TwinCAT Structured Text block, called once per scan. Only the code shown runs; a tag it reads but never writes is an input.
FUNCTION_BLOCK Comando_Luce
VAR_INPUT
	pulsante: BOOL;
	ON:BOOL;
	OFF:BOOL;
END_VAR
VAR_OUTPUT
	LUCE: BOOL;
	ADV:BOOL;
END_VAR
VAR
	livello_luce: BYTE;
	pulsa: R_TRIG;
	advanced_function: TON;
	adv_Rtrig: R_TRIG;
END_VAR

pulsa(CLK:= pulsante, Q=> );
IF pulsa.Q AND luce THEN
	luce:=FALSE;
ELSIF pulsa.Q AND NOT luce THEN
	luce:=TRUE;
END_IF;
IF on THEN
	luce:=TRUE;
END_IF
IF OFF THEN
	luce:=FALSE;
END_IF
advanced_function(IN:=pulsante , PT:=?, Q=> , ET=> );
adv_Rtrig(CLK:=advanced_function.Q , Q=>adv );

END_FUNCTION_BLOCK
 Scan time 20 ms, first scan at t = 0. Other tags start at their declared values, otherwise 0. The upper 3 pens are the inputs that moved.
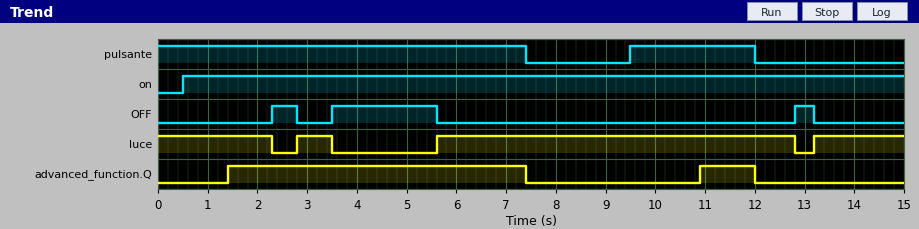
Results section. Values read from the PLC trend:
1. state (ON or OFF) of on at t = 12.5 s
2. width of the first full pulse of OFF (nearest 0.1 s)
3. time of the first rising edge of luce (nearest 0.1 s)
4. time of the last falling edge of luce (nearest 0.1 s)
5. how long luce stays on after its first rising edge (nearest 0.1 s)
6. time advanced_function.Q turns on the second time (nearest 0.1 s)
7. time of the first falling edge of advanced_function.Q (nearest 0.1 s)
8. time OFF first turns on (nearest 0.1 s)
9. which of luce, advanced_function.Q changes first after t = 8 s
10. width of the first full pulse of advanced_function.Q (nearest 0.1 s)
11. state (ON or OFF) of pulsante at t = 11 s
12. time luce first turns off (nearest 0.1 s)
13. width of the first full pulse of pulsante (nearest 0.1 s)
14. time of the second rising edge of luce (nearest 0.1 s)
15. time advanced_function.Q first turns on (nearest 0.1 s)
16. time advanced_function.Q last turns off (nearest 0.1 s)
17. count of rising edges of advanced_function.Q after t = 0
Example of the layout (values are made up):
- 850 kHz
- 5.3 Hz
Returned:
- ON
- 0.5 s
- 2.8 s
- 12.8 s
- 0.7 s
- 10.9 s
- 7.4 s
- 2.3 s
- advanced_function.Q
- 6.0 s
- ON
- 2.3 s
- 2.5 s
- 5.6 s
- 1.4 s
- 12.0 s
- 2
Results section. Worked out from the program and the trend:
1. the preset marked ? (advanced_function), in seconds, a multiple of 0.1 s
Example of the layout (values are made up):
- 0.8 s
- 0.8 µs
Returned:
- 1.4 s
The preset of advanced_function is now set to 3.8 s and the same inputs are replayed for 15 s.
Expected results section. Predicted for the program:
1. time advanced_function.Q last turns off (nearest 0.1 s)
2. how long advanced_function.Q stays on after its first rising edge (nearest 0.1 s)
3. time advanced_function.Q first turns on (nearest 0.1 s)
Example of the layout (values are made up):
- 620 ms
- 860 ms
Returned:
- 7.4 s
- 3.6 s
- 3.8 s
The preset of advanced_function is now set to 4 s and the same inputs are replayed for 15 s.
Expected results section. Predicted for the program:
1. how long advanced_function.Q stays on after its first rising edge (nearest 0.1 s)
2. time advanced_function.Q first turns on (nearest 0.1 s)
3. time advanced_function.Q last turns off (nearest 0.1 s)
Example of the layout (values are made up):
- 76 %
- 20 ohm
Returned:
- 3.4 s
- 4.0 s
- 7.4 s
